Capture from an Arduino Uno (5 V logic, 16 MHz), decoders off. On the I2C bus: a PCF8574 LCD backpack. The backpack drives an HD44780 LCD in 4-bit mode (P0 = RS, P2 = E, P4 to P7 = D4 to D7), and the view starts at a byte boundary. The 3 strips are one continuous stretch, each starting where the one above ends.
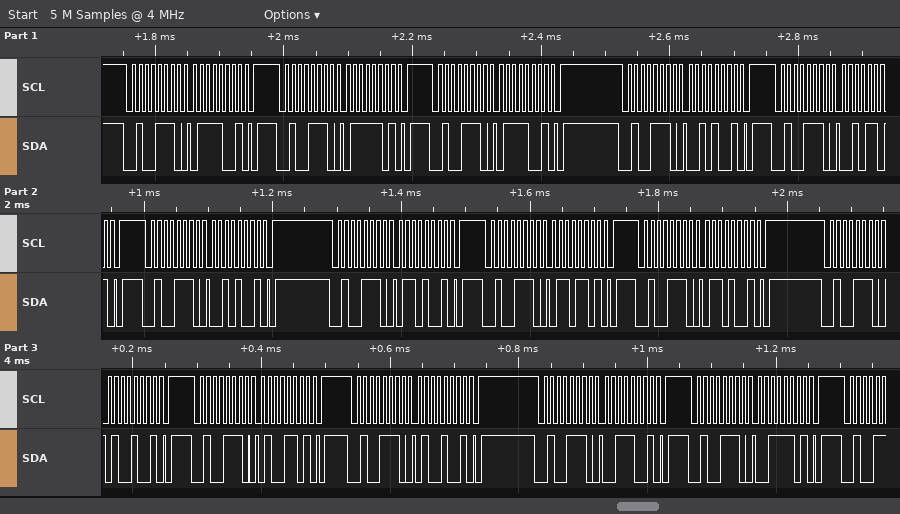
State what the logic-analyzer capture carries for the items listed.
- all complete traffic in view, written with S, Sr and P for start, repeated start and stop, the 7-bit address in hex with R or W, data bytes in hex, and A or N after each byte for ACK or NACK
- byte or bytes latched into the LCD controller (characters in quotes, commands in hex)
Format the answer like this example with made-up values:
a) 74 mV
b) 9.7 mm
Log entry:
a) S 27W A 79 A P S 27W A 7D A P S 27W A 79 A P S 27W A 29 A P S 27W A 2D A P S 27W A 29 A P S 27W A 69 A P S 27W A 6D A P S 27W A 69 A P S 27W A 49 A P S 27W A 4D A P S 27W A 49 A P S 27W A 39 A P S 27W A 3D A P
b) 'r' 'd'
